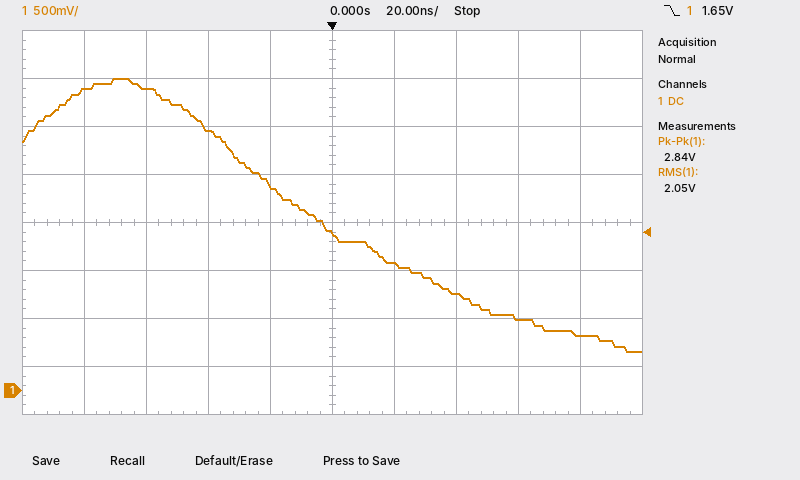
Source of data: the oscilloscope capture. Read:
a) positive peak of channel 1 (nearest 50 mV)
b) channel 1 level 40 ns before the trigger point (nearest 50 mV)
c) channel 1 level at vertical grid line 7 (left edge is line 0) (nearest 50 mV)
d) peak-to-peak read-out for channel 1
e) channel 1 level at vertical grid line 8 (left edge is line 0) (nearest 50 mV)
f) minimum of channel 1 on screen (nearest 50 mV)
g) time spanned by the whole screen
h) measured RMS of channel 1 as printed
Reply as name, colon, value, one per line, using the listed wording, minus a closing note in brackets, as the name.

positive peak of channel 1: 3.25 V
channel 1 level 40 ns before the trigger point: 2.70 V
channel 1 level at vertical grid line 7 (left edge is line 0): 1.00 V
peak-to-peak read-out for channel 1: 2.84 V
channel 1 level at vertical grid line 8 (left edge is line 0): 750 mV
minimum of channel 1 on screen: 400 mV
time spanned by the whole screen: 200 ns
measured RMS of channel 1 as printed: 2.05 V
